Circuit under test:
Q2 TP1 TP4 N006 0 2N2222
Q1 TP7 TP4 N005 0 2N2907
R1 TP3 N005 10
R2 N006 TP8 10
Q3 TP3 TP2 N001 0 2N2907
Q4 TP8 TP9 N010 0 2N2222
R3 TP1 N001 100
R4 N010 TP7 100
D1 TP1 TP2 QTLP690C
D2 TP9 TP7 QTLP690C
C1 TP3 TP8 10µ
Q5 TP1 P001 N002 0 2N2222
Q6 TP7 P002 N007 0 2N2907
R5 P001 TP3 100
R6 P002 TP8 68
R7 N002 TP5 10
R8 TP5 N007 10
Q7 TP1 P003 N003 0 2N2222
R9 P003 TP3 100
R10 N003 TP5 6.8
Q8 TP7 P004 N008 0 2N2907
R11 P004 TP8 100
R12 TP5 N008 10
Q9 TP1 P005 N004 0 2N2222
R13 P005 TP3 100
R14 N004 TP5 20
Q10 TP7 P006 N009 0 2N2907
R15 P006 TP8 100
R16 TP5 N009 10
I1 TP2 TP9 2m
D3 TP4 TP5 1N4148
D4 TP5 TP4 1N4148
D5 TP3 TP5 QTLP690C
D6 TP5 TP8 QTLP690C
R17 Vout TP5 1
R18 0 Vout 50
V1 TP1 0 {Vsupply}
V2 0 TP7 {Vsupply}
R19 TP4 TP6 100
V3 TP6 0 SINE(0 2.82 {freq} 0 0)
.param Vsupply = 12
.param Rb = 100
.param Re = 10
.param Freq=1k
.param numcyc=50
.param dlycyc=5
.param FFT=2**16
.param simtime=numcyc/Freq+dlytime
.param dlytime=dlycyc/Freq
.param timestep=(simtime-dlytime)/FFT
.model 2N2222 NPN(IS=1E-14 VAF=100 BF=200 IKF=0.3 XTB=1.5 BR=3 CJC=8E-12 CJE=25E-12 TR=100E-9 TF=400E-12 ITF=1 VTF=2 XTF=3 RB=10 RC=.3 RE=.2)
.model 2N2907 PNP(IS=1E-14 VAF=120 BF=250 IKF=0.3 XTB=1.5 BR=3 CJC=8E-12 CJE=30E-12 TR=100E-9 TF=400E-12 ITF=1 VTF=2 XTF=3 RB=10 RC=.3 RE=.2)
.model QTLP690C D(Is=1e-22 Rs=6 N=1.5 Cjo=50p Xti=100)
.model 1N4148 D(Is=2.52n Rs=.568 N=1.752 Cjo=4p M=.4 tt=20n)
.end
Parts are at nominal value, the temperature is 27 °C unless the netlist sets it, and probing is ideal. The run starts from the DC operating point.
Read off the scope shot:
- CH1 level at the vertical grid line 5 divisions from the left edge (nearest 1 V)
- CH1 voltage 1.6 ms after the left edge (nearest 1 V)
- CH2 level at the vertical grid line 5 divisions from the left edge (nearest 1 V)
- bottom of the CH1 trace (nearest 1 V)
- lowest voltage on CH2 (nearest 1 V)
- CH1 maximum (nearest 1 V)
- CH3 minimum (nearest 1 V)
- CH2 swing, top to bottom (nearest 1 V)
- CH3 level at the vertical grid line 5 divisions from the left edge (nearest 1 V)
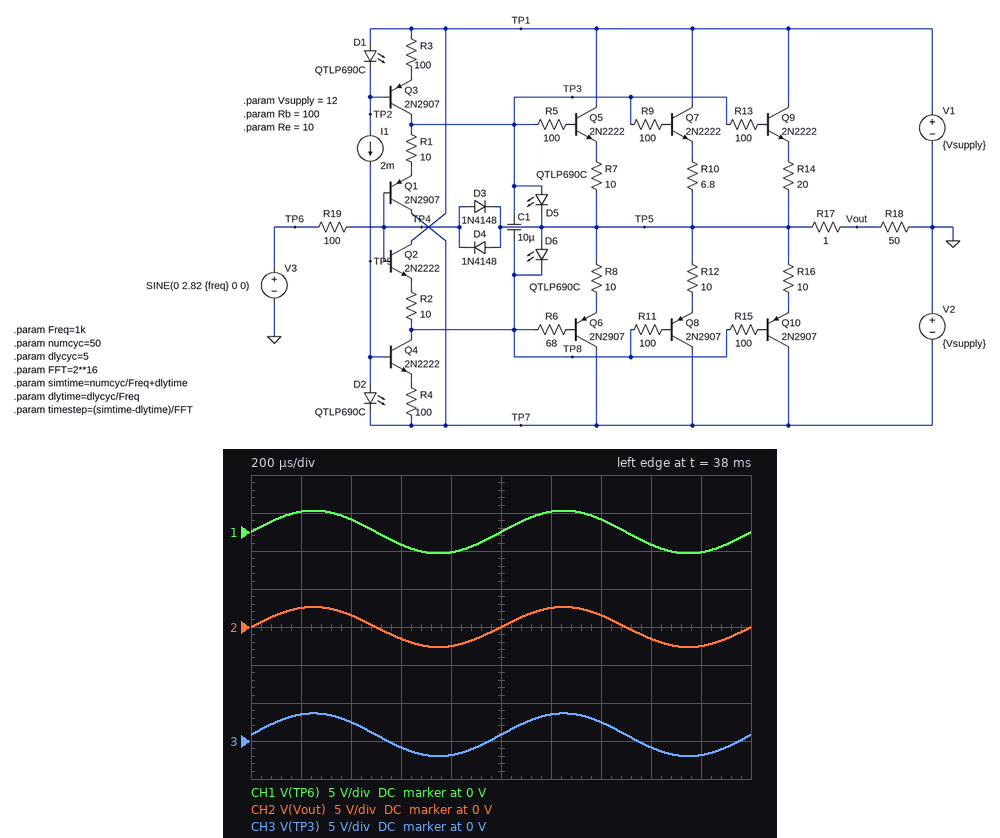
0 V
-2 V
0 V
-3 V
-3 V
3 V
-2 V
5 V
1 V
